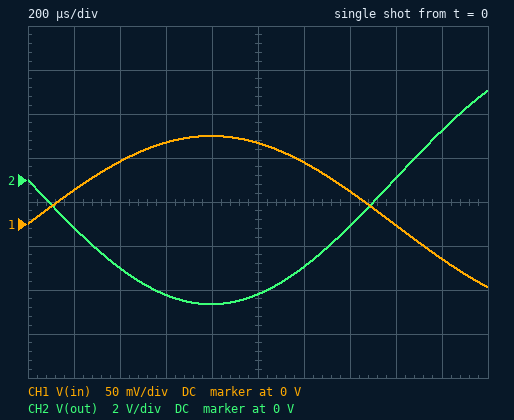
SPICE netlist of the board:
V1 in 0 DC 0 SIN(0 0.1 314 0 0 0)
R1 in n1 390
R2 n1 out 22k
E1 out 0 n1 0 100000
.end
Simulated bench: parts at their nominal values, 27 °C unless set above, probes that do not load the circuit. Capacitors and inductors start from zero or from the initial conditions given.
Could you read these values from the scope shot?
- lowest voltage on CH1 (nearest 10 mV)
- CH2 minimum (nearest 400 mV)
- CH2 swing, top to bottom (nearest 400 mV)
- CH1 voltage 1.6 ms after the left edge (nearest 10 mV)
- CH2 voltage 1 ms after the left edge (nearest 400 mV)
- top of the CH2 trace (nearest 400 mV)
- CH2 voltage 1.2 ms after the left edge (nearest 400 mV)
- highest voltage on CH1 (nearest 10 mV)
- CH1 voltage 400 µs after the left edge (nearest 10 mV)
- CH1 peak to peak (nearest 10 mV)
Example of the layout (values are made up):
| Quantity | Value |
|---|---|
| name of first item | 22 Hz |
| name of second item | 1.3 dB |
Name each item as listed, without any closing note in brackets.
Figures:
| Quantity | Value |
|---|---|
| lowest voltage on CH1 | -70 mV |
| CH2 minimum | -5.6 V |
| CH2 swing, top to bottom | 9.6 V |
| CH1 voltage 1.6 ms after the left edge | 0 V |
| CH2 voltage 1 ms after the left edge | -5.2 V |
| top of the CH2 trace | 4.0 V |
| CH2 voltage 1.2 ms after the left edge | -4.0 V |
| highest voltage on CH1 | 100 mV |
| CH1 voltage 400 µs after the left edge | 70 mV |
| CH1 peak to peak | 170 mV |
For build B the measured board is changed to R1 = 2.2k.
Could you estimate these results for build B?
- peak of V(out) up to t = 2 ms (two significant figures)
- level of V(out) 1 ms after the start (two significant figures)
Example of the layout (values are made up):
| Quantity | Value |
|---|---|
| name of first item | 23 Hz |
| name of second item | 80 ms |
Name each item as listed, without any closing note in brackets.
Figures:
| Quantity | Value |
|---|---|
| peak of V(out) up to t = 2 ms | 720 mV |
| level of V(out) 1 ms after the start | -920 mV |
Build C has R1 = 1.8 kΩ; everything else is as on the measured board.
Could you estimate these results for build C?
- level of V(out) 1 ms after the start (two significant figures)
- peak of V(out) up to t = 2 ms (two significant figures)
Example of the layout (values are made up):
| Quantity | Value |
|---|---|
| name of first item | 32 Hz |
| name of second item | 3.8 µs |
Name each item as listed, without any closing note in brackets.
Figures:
| Quantity | Value |
|---|---|
| level of V(out) 1 ms after the start | -1.1 V |
| peak of V(out) up to t = 2 ms | 880 mV |
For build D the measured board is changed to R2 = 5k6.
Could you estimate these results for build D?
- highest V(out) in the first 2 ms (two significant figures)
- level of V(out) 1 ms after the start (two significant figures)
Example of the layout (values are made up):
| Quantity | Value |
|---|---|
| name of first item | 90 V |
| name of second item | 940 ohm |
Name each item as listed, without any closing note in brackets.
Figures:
| Quantity | Value |
|---|---|
| highest V(out) in the first 2 ms | 1.0 V |
| level of V(out) 1 ms after the start | -1.3 V |
